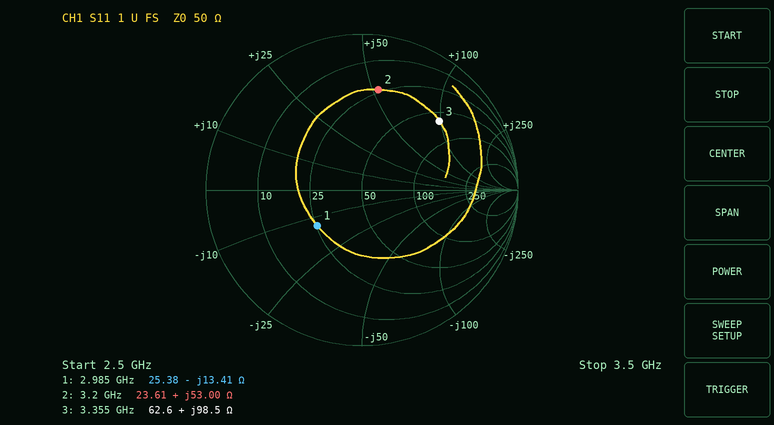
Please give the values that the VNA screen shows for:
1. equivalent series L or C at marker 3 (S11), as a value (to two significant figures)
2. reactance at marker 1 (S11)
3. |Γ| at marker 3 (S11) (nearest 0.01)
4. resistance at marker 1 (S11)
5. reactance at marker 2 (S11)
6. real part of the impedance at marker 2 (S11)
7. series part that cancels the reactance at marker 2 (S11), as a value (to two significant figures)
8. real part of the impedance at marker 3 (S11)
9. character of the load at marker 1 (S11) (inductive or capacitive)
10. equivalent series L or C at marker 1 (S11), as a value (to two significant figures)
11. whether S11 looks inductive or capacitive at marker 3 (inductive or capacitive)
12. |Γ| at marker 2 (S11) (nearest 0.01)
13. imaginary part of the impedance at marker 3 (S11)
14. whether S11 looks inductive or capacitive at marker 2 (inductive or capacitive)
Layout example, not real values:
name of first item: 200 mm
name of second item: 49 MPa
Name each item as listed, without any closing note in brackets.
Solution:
equivalent series L or C at marker 3 (S11), as a value: 4.7 nH
reactance at marker 1: -13.41 Ω
|Γ| at marker 3 (S11): 0.66
resistance at marker 1: 25.38 Ω
reactance at marker 2: +53.00 Ω
real part of the impedance at marker 2: 23.61 Ω
series part that cancels the reactance at marker 2 (S11), as a value: 940 fF
real part of the impedance at marker 3: 62.6 Ω
character of the load at marker 1 (S11): capacitive
equivalent series L or C at marker 1 (S11), as a value: 4.0 pF
whether S11 looks inductive or capacitive at marker 3: inductive
|Γ| at marker 2 (S11): 0.65
imaginary part of the impedance at marker 3: +98.5 Ω
whether S11 looks inductive or capacitive at marker 2: inductive
